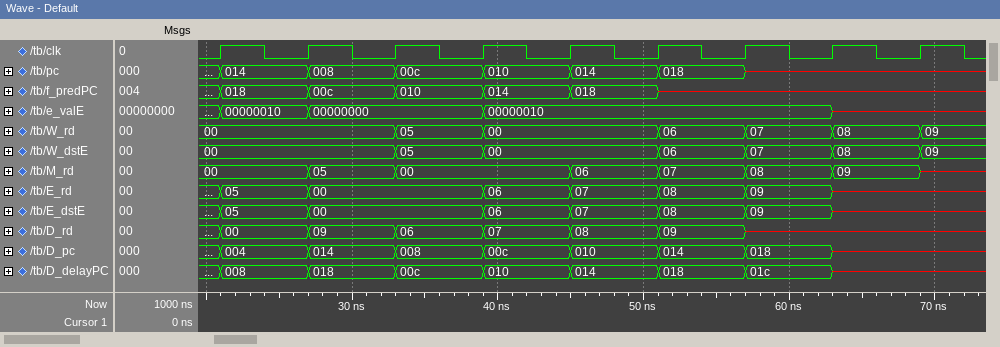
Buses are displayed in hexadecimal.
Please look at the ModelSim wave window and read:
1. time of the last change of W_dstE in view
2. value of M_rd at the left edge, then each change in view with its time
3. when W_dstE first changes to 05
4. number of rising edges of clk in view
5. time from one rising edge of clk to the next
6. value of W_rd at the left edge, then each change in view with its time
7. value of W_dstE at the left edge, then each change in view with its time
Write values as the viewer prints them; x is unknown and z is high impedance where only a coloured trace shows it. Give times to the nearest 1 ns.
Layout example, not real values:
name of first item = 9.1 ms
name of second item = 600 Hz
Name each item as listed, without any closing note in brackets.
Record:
time of the last change of W_dstE in view = 69 ns
value of M_rd at the left edge, then each change in view with its time = 00, 05 at 27 ns, 00 at 33 ns, 06 at 45 ns, 07 at 51 ns, 08 at 57 ns, 09 at 63 ns, x at 69 ns
when W_dstE first changes to 05 = 33 ns
number of rising edges of clk in view = 9
time from one rising edge of clk to the next = 6 ns
value of W_rd at the left edge, then each change in view with its time = 00, 05 at 33 ns, 00 at 39 ns, 06 at 51 ns, 07 at 57 ns, 08 at 63 ns, 09 at 69 ns
value of W_dstE at the left edge, then each change in view with its time = 00, 05 at 33 ns, 00 at 39 ns, 06 at 51 ns, 07 at 57 ns, 08 at 63 ns, 09 at 69 ns
